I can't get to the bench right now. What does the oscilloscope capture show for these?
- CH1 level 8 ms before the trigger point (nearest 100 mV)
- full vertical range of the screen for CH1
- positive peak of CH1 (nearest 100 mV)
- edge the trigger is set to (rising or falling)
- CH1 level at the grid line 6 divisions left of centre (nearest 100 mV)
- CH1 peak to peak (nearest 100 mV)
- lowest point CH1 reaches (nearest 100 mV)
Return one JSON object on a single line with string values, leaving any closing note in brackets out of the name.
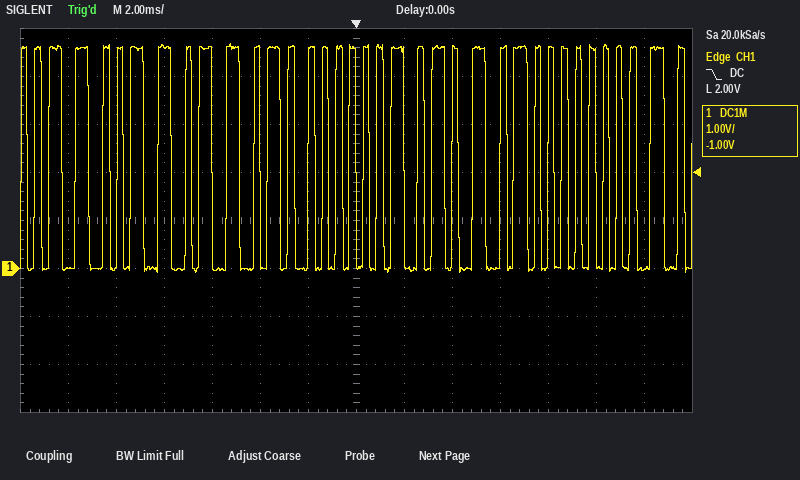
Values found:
{"CH1 level 8 ms before the trigger point": "4.6 V", "full vertical range of the screen for CH1": "8 V", "positive peak of CH1": "4.7 V", "edge the trigger is set to": "falling", "CH1 level at the grid line 6 divisions left of centre": "0.0 V", "CH1 peak to peak": "4.8 V", "lowest point CH1 reaches": "-100 mV"}
